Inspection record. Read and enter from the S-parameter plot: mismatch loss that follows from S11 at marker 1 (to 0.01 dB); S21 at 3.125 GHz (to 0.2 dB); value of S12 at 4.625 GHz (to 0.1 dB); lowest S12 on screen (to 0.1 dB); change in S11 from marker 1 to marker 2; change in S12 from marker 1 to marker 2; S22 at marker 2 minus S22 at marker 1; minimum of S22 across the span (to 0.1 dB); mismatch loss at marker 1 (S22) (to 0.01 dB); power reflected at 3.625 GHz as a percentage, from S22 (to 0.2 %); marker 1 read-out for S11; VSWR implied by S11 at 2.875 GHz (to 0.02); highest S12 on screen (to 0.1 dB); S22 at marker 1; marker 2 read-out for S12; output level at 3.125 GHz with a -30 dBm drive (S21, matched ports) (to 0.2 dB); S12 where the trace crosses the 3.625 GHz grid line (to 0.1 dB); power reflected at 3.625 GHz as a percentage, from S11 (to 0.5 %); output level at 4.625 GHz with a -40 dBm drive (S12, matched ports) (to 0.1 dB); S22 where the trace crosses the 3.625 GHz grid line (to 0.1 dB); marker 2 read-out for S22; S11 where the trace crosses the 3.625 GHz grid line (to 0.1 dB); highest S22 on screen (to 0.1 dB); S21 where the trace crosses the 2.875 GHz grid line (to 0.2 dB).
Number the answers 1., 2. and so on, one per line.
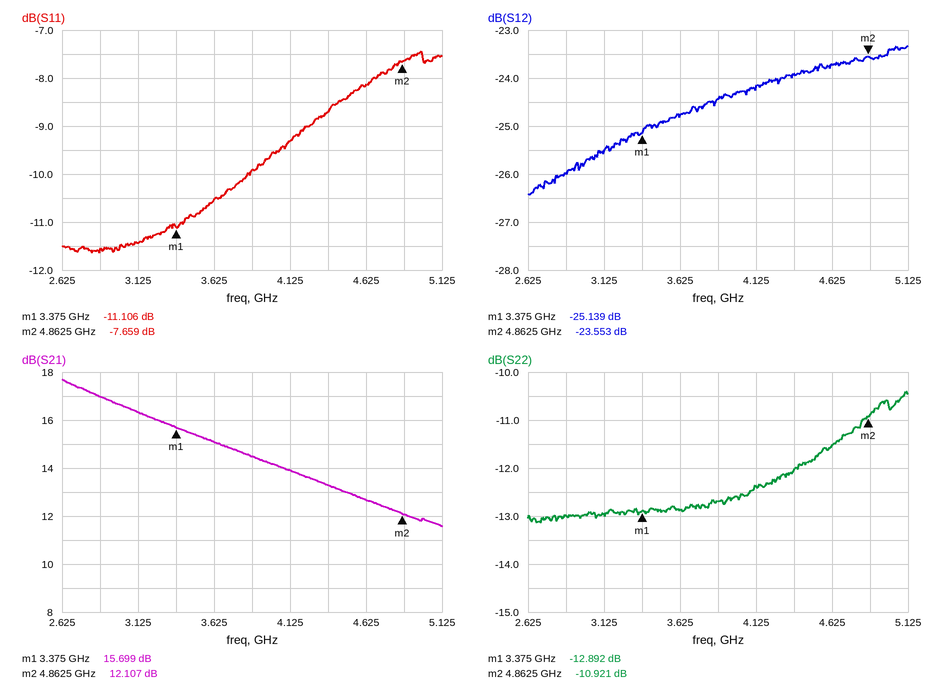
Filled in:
1. 0.35 dB
2. 16.4 dB
3. -23.7 dB
4. -26.4 dB
5. 3.447 dB
6. 1.586 dB
7. 1.971 dB
8. -13.1 dB
9. 0.23 dB
10. 5.2 %
11. -11.106 dB
12. 1.72
13. -23.3 dB
14. -12.892 dB
15. -23.553 dB
16. -13.6 dBm
17. -24.8 dB
18. 9.0 %
19. -63.7 dBm
20. -12.9 dB
21. -10.921 dB
22. -10.5 dB
23. -10.4 dB
24. 17.0 dB
